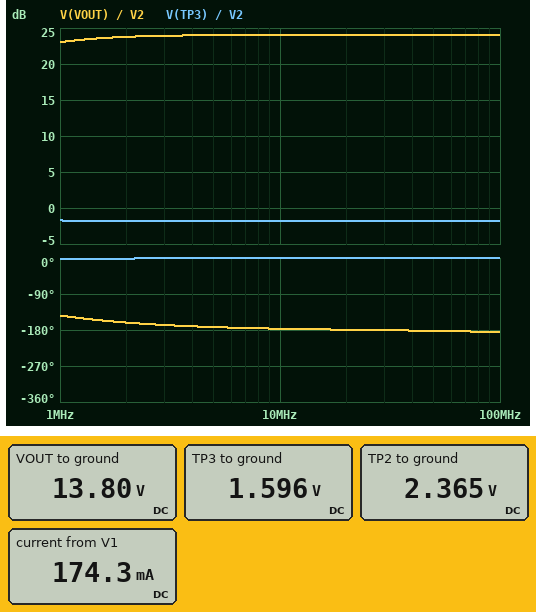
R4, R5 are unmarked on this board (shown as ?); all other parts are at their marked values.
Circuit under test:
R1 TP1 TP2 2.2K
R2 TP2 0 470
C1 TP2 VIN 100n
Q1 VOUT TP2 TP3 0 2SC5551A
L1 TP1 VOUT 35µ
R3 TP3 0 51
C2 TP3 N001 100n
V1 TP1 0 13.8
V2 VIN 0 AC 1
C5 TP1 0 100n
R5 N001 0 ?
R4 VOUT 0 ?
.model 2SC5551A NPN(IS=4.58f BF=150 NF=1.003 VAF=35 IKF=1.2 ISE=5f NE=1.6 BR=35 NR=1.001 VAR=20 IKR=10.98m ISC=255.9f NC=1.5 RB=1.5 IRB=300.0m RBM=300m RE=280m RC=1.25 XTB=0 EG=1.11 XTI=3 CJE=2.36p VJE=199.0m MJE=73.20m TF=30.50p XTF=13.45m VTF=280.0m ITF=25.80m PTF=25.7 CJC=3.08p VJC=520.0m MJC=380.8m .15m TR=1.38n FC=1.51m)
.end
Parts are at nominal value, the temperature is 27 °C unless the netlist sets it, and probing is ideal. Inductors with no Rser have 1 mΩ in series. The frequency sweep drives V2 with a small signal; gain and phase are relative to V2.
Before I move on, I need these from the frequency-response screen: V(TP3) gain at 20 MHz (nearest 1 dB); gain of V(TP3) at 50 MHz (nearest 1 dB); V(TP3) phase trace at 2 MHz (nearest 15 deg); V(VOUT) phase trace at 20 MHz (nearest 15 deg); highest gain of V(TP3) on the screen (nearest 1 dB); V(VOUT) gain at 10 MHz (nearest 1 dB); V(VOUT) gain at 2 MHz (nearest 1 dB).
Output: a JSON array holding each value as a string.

["-2 dB", "-2 dB", "0 deg", "-180 deg", "-2 dB", "24 dB", "24 dB"]
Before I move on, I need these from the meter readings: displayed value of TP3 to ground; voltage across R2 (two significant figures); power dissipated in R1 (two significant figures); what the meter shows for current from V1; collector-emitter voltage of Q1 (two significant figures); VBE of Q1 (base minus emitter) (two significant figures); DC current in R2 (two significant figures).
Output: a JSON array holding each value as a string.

["1.596 V", "2.4 V", "59 mW", "174.3 mA", "12 V", "770 mV", "5.0 mA"]
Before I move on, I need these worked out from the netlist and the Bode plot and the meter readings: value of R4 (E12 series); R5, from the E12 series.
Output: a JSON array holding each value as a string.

["100 Ω", "5.6 Ω"]
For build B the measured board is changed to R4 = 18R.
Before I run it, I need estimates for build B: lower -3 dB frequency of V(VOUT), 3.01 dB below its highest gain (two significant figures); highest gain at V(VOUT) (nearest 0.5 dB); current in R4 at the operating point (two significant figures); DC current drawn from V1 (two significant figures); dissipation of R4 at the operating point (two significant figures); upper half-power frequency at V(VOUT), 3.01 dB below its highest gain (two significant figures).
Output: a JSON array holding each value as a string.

["260 kHz", "9.0 dB", "770 mA", "800 mA", "11 W", "5.8 GHz"]
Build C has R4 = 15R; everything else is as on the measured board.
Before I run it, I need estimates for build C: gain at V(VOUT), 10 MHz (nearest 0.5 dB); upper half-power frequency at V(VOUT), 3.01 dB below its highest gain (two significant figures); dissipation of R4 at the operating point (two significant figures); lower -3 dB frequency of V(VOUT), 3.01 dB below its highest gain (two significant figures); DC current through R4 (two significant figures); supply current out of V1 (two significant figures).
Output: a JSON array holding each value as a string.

["7.5 dB", "6.6 GHz", "13 W", "250 kHz", "920 mA", "960 mA"]
